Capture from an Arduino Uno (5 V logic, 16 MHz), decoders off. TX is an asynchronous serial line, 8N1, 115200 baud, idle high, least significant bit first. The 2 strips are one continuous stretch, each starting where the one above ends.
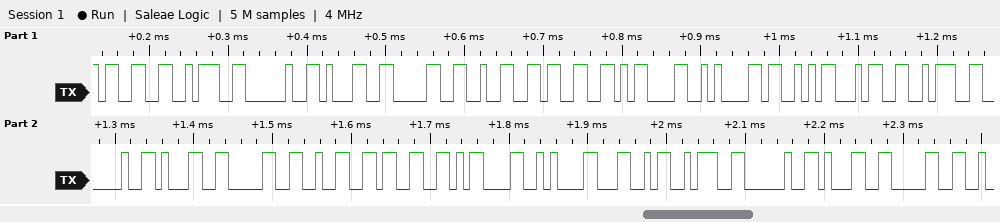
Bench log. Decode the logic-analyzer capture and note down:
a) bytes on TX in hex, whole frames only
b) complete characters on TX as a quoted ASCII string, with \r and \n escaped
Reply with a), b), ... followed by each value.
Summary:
a) 33 3A 20 31 30 32 33 0D 0A 53 34 3A 20 31 30 32 33 0D 0A 4C 3A 20 31 30
b) "3: 1023\r\nS4: 1023\r\nL: 10"
